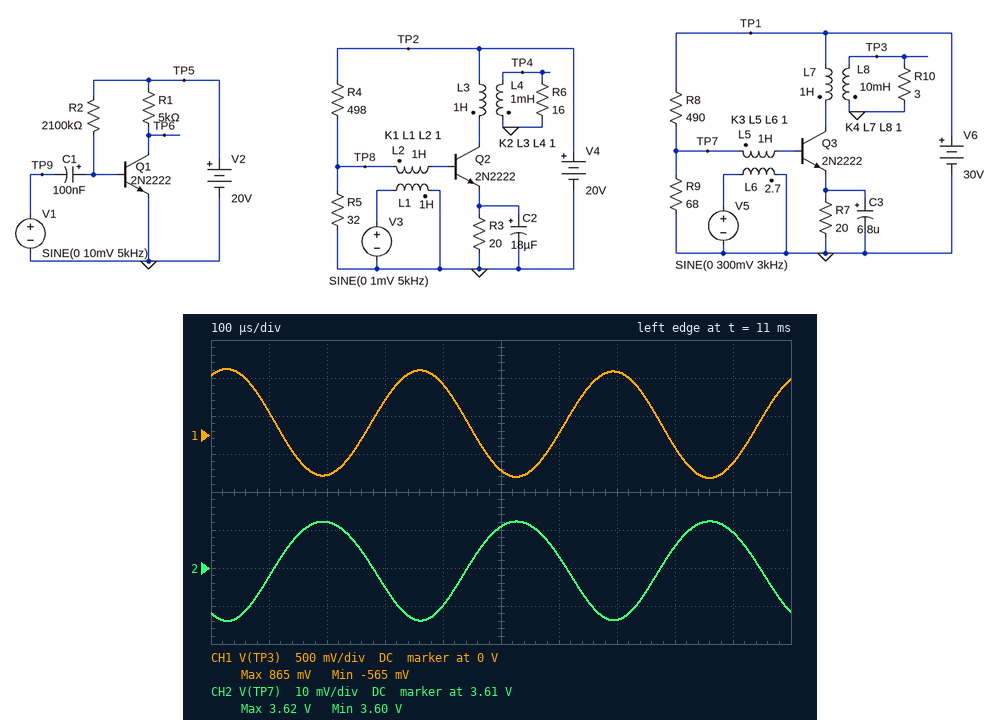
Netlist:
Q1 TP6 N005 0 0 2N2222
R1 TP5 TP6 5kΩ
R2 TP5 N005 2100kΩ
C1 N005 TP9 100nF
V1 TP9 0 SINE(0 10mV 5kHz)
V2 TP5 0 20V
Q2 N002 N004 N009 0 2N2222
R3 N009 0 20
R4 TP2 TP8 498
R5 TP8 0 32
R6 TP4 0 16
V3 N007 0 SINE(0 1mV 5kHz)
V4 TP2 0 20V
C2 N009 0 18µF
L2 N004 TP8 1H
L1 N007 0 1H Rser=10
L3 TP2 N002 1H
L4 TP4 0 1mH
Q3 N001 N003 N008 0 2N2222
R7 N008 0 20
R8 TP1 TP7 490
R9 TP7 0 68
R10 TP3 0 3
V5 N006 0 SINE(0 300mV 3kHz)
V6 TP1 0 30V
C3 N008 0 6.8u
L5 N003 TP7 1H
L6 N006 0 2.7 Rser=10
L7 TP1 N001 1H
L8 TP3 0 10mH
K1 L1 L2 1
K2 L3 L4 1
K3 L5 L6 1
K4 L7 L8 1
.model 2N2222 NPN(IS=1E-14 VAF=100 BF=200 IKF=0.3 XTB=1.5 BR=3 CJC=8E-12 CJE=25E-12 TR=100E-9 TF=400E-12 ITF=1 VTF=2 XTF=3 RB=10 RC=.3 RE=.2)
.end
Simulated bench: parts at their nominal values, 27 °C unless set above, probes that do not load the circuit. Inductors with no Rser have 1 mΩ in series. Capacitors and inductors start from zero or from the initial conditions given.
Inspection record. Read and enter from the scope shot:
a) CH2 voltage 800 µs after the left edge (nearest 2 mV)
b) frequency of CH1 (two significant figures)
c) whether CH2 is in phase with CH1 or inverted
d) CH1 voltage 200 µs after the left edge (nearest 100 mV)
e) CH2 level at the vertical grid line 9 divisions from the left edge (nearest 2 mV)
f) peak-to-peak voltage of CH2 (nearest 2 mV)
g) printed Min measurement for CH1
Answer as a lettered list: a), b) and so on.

a) 3.616 V
b) 3.0 kHz
c) inverted
d) -500 mV
e) 3.620 V
f) 26 mV
g) -565 mV
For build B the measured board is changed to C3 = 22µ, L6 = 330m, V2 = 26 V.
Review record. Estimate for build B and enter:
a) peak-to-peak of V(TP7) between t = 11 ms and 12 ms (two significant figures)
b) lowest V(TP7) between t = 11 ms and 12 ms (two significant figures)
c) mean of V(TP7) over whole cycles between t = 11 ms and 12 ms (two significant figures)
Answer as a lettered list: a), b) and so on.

a) 310 mV
b) 3.3 V
c) 3.5 V
